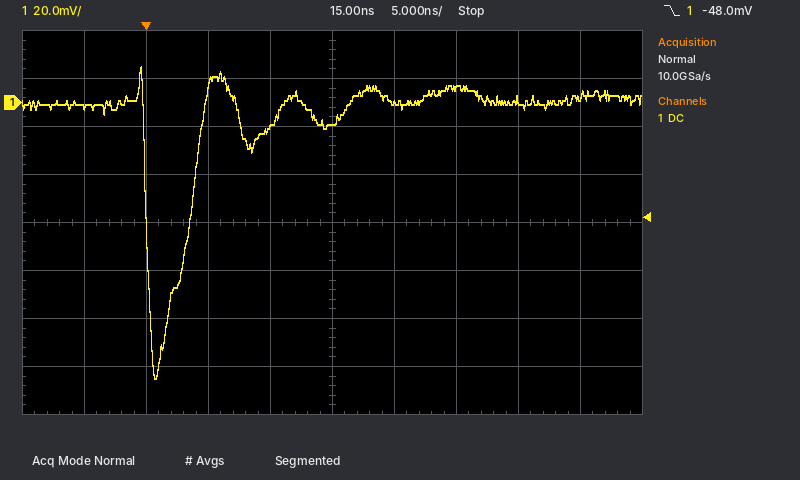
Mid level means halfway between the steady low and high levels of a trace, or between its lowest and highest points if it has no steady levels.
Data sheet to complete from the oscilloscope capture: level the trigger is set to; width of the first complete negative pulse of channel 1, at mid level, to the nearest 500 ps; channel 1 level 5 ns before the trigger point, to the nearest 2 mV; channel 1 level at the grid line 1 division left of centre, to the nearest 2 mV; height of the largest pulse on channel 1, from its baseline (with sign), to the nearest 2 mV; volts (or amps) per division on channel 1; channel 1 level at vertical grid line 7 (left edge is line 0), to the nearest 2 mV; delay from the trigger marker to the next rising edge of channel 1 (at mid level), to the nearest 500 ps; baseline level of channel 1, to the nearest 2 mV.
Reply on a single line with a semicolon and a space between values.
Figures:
-48.0 mV; 3.5 ns; -2 mV; -10 mV; -114 mV; 20 mV; 6 mV; 3.5 ns; 0 mV
